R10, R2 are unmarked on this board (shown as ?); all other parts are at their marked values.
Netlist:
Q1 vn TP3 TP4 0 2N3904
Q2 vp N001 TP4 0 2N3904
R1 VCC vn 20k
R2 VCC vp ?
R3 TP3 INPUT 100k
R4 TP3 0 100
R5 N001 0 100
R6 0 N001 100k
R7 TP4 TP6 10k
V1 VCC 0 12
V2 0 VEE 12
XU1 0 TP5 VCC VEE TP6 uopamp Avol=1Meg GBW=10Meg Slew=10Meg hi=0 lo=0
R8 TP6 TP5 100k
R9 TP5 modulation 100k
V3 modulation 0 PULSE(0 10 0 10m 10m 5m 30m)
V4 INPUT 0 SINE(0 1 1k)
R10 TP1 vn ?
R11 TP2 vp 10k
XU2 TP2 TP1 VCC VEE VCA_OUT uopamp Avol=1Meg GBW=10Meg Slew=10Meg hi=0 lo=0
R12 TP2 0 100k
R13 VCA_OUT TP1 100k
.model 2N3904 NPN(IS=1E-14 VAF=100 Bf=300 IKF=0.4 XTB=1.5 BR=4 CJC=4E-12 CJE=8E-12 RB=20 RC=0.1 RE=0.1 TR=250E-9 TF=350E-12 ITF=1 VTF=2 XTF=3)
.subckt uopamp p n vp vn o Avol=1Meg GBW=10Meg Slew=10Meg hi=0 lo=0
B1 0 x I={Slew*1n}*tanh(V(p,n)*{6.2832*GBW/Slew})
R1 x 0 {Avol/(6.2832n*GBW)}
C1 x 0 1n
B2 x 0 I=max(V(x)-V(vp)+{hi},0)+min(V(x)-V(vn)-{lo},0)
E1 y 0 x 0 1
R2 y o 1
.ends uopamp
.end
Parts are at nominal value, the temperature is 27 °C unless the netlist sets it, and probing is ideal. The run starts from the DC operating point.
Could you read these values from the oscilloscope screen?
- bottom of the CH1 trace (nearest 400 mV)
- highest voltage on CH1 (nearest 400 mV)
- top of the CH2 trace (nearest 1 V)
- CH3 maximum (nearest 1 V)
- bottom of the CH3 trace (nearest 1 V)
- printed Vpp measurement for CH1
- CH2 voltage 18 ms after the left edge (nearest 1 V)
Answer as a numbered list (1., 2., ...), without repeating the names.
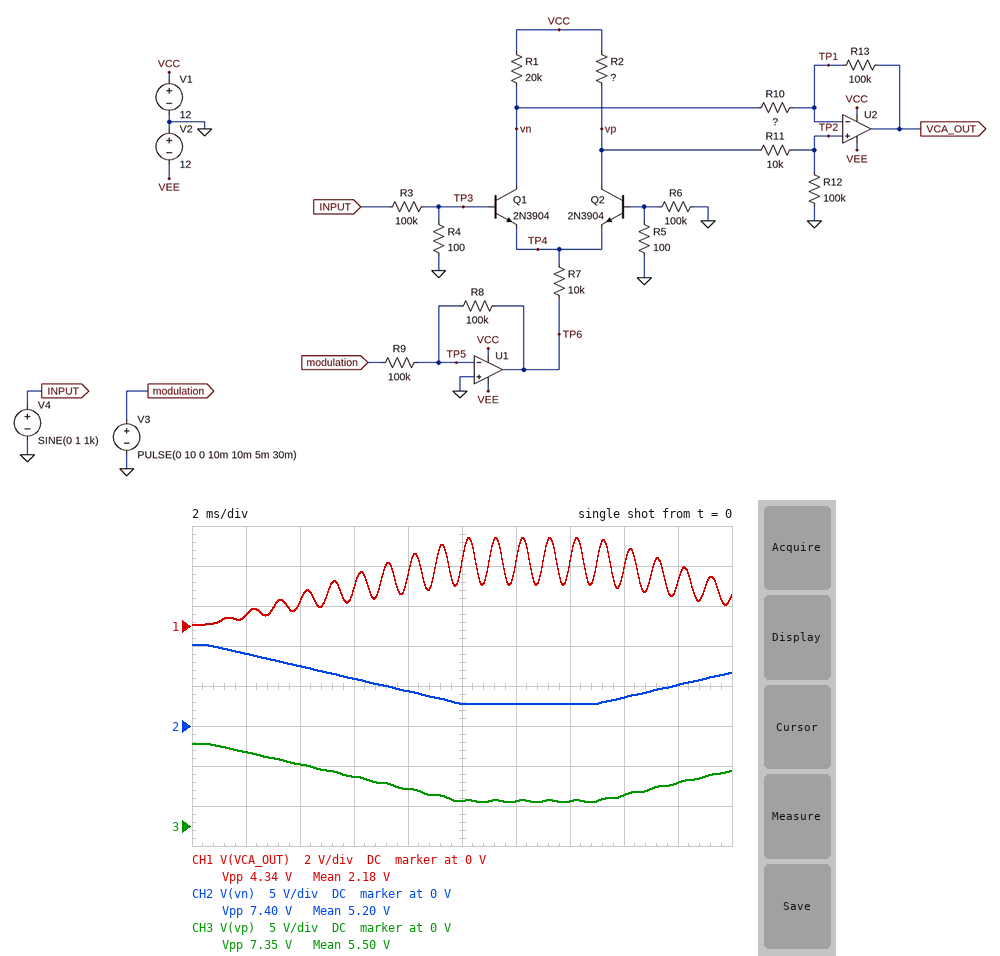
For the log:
1. 0 V
2. 4.4 V
3. 10 V
4. 10 V
5. 3 V
6. 4.34 V
7. 5 V
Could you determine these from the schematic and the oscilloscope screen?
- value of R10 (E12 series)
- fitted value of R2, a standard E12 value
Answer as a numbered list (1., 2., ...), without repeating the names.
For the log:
1. 8.2 kΩ
2. 18 kΩ
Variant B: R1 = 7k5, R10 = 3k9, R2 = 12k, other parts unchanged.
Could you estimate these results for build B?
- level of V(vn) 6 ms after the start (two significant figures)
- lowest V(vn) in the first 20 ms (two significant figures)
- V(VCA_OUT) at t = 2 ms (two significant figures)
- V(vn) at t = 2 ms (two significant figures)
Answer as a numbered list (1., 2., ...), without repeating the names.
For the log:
1. 8.5 V
2. 7.0 V
3. -11 V
4. 9.9 V
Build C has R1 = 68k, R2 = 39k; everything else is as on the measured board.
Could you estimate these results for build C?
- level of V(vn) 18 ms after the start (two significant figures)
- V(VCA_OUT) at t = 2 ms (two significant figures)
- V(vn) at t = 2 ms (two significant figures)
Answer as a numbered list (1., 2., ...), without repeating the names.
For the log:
1. -630 mV
2. 4.9 V
3. 6.3 V
